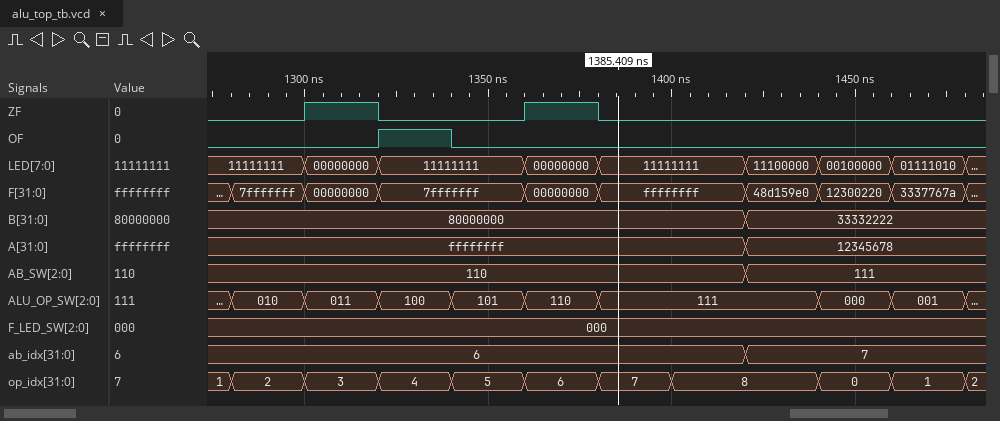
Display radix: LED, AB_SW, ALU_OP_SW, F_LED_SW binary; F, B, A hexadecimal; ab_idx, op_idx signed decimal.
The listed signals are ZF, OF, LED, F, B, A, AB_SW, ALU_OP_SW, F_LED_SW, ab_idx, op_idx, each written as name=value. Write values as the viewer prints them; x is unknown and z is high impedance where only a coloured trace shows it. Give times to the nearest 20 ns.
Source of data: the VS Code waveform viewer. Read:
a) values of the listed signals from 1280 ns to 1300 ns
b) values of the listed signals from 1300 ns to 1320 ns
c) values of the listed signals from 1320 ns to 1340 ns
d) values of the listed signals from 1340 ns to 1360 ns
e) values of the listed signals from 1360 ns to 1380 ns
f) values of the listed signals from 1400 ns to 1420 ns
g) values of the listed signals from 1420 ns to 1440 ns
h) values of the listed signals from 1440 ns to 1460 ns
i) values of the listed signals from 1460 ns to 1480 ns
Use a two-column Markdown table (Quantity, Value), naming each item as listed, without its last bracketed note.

| Quantity | Value |
|---|---|
| values of the listed signals from 1280 ns to 1300 ns | ZF=0, OF=0, LED=11111111, F=7fffffff, B=80000000, A=ffffffff, AB_SW=110, ALU_OP_SW=010, F_LED_SW=000, ab_idx=6, op_idx=2 |
| values of the listed signals from 1300 ns to 1320 ns | ZF=1, OF=0, LED=00000000, F=00000000, B=80000000, A=ffffffff, AB_SW=110, ALU_OP_SW=011, F_LED_SW=000, ab_idx=6, op_idx=3 |
| values of the listed signals from 1320 ns to 1340 ns | ZF=0, OF=1, LED=11111111, F=7fffffff, B=80000000, A=ffffffff, AB_SW=110, ALU_OP_SW=100, F_LED_SW=000, ab_idx=6, op_idx=4 |
| values of the listed signals from 1340 ns to 1360 ns | ZF=0, OF=0, LED=11111111, F=7fffffff, B=80000000, A=ffffffff, AB_SW=110, ALU_OP_SW=101, F_LED_SW=000, ab_idx=6, op_idx=5 |
| values of the listed signals from 1360 ns to 1380 ns | ZF=1, OF=0, LED=00000000, F=00000000, B=80000000, A=ffffffff, AB_SW=110, ALU_OP_SW=110, F_LED_SW=000, ab_idx=6, op_idx=6 |
| values of the listed signals from 1400 ns to 1420 ns | ZF=0, OF=0, LED=11111111, F=ffffffff, B=80000000, A=ffffffff, AB_SW=110, ALU_OP_SW=111, F_LED_SW=000, ab_idx=6, op_idx=8 |
| values of the listed signals from 1420 ns to 1440 ns | ZF=0, OF=0, LED=11100000, F=48d159e0, B=33332222, A=12345678, AB_SW=111, ALU_OP_SW=111, F_LED_SW=000, ab_idx=7, op_idx=8 |
| values of the listed signals from 1440 ns to 1460 ns | ZF=0, OF=0, LED=00100000, F=12300220, B=33332222, A=12345678, AB_SW=111, ALU_OP_SW=000, F_LED_SW=000, ab_idx=7, op_idx=0 |
| values of the listed signals from 1460 ns to 1480 ns | ZF=0, OF=0, LED=01111010, F=3337767a, B=33332222, A=12345678, AB_SW=111, ALU_OP_SW=001, F_LED_SW=000, ab_idx=7, op_idx=1 |
